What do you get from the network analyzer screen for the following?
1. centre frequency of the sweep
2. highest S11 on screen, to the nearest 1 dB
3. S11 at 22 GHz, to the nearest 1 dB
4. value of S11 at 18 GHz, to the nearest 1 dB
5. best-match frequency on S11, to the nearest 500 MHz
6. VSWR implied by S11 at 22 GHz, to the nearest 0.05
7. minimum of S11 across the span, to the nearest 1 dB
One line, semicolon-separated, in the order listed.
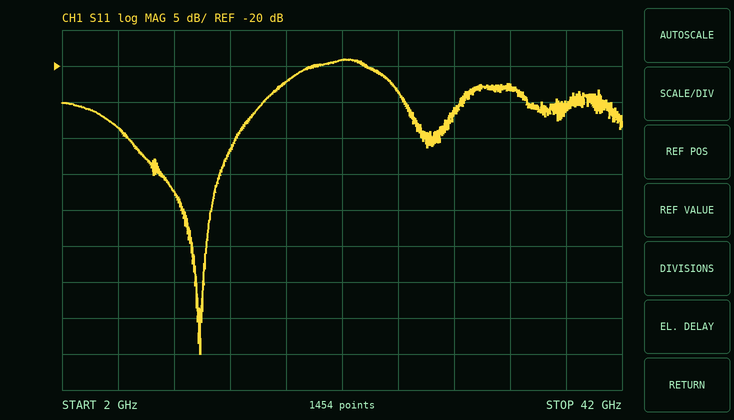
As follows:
22 GHz; -19 dB; -19 dB; -22 dB; 12.0 GHz; 1.25; -60 dB
